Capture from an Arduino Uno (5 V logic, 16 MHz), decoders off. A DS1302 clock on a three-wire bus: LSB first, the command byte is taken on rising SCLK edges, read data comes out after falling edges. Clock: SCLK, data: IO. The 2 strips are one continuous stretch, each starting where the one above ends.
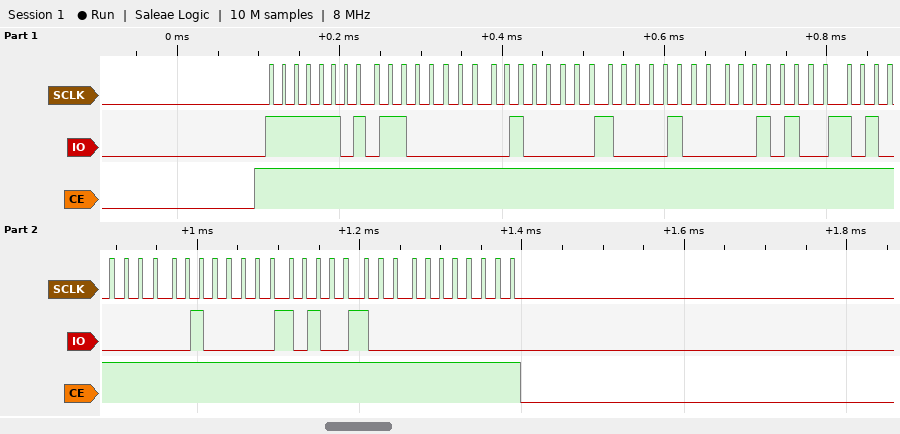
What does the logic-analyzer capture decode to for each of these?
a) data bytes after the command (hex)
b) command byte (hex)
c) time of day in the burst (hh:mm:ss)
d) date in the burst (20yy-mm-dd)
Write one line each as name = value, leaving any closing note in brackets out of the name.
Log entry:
data bytes after the command = 06 04 21 28 05 04 25 00
command byte = 0xBF
time of day in the burst = 21:04:06
date in the burst = 2025-05-28
